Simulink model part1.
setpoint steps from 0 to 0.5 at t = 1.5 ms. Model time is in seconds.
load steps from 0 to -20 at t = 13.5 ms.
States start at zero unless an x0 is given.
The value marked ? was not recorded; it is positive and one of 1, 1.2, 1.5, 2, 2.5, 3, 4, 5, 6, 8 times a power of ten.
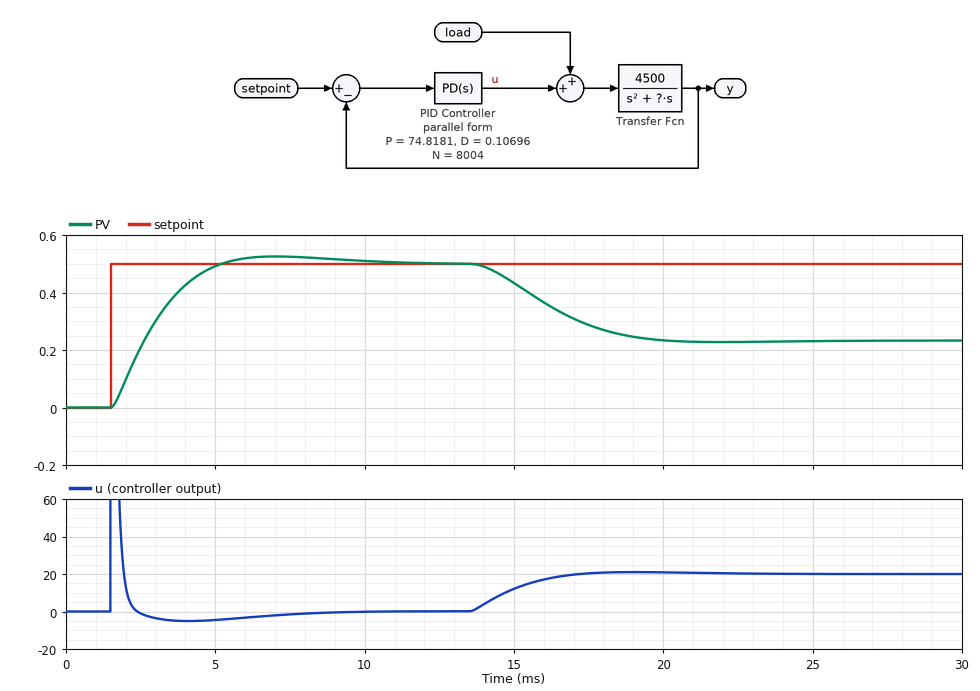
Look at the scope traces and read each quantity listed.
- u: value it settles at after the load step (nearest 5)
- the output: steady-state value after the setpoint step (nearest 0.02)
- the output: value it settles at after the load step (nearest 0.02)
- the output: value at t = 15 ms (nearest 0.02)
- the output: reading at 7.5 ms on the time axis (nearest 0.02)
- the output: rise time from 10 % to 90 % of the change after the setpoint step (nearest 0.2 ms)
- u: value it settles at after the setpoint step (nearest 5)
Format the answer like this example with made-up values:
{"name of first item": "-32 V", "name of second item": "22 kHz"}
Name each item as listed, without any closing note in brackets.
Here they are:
{"u: value it settles at after the load step": "20", "the output: steady-state value after the setpoint step": "0.50", "the output: value it settles at after the load step": "0.24", "the output: value at t = 15 ms": "0.44", "the output: reading at 7.5 ms on the time axis": "0.52", "the output: rise time from 10 % to 90 % of the change after the setpoint step": "2.4 ms", "u: value it settles at after the setpoint step": "0"}
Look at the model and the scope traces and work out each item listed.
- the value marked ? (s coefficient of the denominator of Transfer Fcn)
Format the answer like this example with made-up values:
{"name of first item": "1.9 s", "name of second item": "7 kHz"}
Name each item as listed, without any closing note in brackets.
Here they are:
{"the value marked ?": "400"}
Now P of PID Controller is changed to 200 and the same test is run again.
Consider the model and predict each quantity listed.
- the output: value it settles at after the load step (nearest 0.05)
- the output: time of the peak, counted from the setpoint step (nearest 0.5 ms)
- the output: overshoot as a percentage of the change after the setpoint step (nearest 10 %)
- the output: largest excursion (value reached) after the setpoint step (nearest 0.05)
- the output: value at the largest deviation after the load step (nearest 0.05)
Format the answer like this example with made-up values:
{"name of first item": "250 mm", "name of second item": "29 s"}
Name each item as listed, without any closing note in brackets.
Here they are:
{"the output: value it settles at after the load step": "0.40", "the output: time of the peak, counted from the setpoint step": "3.0 ms", "the output: overshoot as a percentage of the change after the setpoint step": "20 %", "the output: largest excursion (value reached) after the setpoint step": "0.60", "the output: value at the largest deviation after the load step": "0.40"}
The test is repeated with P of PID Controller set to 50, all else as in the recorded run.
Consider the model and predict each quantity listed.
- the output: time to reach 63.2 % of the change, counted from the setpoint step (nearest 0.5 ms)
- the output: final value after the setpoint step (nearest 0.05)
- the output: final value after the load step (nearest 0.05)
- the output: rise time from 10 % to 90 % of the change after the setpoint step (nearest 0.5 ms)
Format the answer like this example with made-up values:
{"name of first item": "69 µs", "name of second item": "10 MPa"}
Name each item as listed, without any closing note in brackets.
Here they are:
{"the output: time to reach 63.2 % of the change, counted from the setpoint step": "2.0 ms", "the output: final value after the setpoint step": "0.50", "the output: final value after the load step": "0.10", "the output: rise time from 10 % to 90 % of the change after the setpoint step": "3.5 ms"}
